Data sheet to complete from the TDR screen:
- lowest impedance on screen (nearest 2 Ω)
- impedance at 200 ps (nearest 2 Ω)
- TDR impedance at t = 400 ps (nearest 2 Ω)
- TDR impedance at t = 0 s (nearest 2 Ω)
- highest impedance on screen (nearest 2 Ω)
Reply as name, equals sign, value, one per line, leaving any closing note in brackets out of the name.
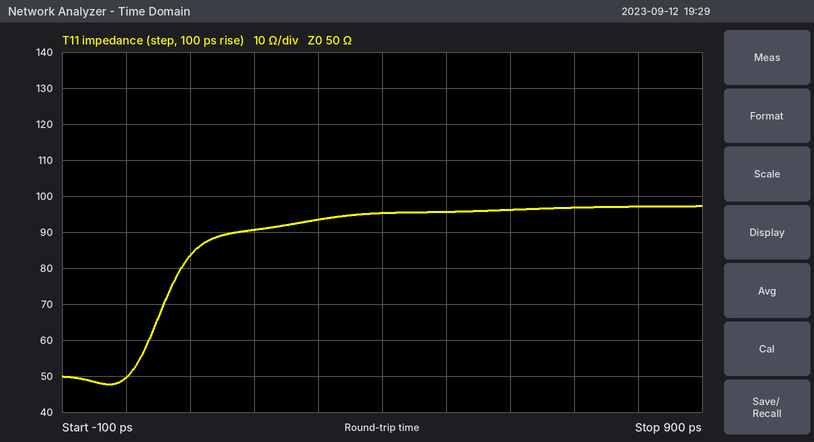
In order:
lowest impedance on screen = 48 Ω
impedance at 200 ps = 90 Ω
TDR impedance at t = 400 ps = 96 Ω
TDR impedance at t = 0 s = 50 Ω
highest impedance on screen = 98 Ω
